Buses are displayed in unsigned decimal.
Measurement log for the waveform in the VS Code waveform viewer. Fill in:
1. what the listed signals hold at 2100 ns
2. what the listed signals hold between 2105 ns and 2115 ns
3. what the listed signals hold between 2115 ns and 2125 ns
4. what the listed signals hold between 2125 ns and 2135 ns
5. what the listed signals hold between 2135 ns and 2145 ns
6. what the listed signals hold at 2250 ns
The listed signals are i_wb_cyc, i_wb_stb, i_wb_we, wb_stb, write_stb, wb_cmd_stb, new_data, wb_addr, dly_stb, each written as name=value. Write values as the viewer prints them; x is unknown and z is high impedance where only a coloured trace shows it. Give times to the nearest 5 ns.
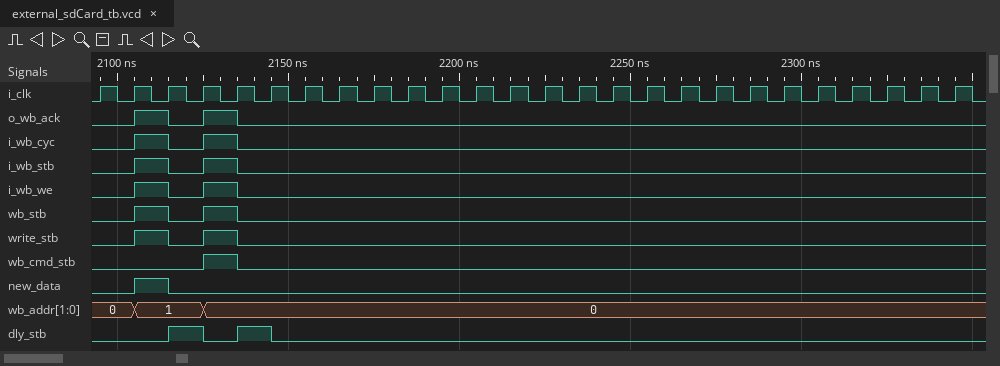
i_wb_cyc=0, i_wb_stb=0, i_wb_we=0, wb_stb=0, write_stb=0, wb_cmd_stb=0, new_data=0, wb_addr=0, dly_stb=0
i_wb_cyc=1, i_wb_stb=1, i_wb_we=1, wb_stb=1, write_stb=1, wb_cmd_stb=0, new_data=1, wb_addr=1, dly_stb=0
i_wb_cyc=0, i_wb_stb=0, i_wb_we=0, wb_stb=0, write_stb=0, wb_cmd_stb=0, new_data=0, wb_addr=1, dly_stb=1
i_wb_cyc=1, i_wb_stb=1, i_wb_we=1, wb_stb=1, write_stb=1, wb_cmd_stb=1, new_data=0, wb_addr=0, dly_stb=0
i_wb_cyc=0, i_wb_stb=0, i_wb_we=0, wb_stb=0, write_stb=0, wb_cmd_stb=0, new_data=0, wb_addr=0, dly_stb=1
i_wb_cyc=0, i_wb_stb=0, i_wb_we=0, wb_stb=0, write_stb=0, wb_cmd_stb=0, new_data=0, wb_addr=0, dly_stb=0
